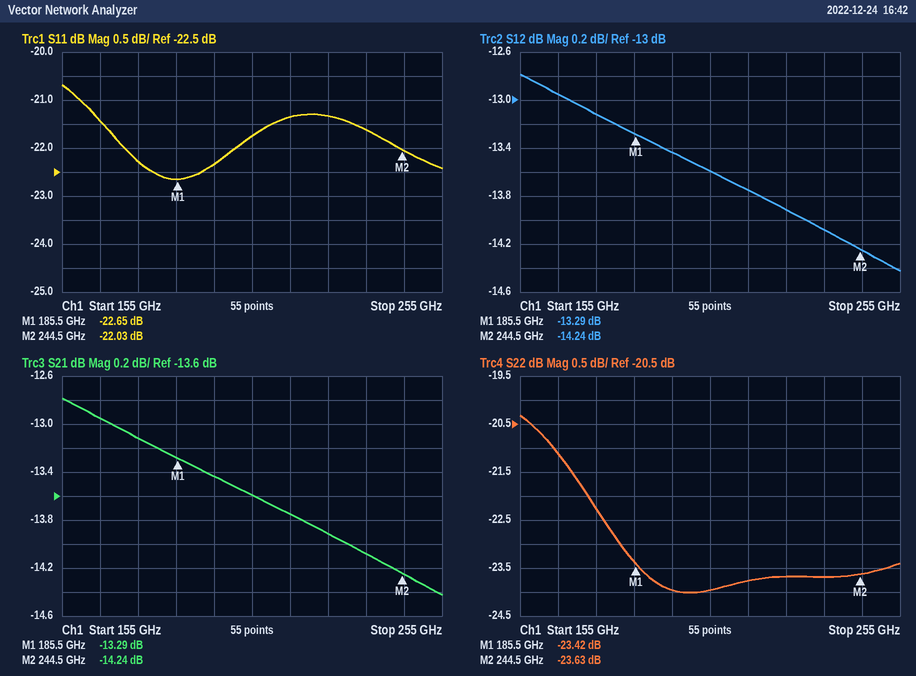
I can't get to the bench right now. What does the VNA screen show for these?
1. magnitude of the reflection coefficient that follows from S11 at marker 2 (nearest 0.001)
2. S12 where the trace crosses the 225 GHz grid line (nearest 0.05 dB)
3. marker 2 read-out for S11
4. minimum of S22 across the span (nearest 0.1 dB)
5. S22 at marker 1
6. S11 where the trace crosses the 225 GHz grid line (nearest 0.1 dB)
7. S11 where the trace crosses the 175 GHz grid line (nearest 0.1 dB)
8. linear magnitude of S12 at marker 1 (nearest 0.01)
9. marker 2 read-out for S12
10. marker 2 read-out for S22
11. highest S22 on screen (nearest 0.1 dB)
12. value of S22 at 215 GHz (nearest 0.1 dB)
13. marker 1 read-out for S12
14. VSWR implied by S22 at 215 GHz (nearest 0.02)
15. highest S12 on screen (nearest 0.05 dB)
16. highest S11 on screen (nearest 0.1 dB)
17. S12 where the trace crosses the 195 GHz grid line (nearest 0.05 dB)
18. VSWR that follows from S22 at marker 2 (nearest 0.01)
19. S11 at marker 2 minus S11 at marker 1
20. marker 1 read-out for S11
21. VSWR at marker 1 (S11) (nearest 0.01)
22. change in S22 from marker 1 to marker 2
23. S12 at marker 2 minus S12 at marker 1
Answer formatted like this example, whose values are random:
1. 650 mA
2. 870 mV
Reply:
1. 0.079
2. -13.90 dB
3. -22.03 dB
4. -24.0 dB
5. -23.42 dB
6. -21.3 dB
7. -22.3 dB
8. 0.22
9. -14.24 dB
10. -23.63 dB
11. -20.3 dB
12. -23.8 dB
13. -13.29 dB
14. 1.14
15. -12.80 dB
16. -20.7 dB
17. -13.45 dB
18. 1.14
19. 0.62 dB
20. -22.65 dB
21. 1.16
22. -0.21 dB
23. -0.95 dB
